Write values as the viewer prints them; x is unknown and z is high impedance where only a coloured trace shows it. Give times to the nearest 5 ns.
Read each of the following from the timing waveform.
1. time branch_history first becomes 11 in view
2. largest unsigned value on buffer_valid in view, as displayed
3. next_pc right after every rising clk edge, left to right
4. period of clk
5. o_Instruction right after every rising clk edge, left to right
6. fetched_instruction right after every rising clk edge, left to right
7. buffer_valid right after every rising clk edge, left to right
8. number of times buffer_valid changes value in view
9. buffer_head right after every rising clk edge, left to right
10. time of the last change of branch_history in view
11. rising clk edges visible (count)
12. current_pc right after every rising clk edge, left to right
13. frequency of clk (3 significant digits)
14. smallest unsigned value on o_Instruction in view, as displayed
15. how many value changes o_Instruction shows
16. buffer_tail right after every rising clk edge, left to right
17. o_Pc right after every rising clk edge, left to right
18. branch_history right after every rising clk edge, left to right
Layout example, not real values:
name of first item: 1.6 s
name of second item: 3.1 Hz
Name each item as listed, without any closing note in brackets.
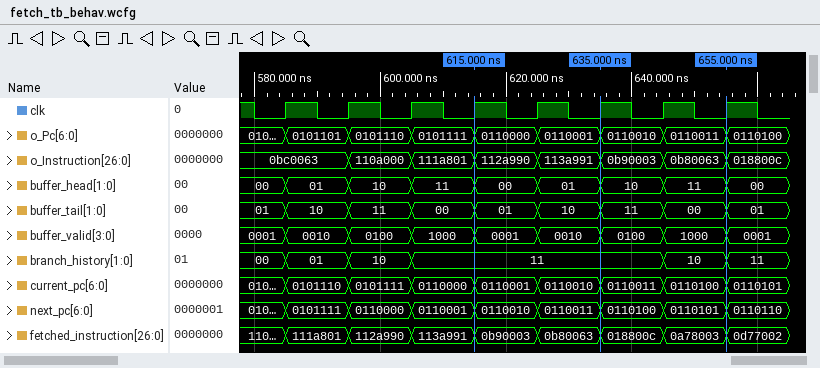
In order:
time branch_history first becomes 11 in view: 605 ns
largest unsigned value on buffer_valid in view, as displayed: 1000
next_pc right after every rising clk edge, left to right: 0101111, 0110000, 0110001, 0110010, 0110011, 0110100, 0110101, 0110110
period of clk: 10 ns
o_Instruction right after every rising clk edge, left to right: 0bc0063, 110a000, 111a801, 112a990, 113a991, 0b90003, 0b80063, 018800c
fetched_instruction right after every rising clk edge, left to right: 111a801, 112a990, 113a991, 0b90003, 0b80063, 018800c, 0a78003, 0d77002
buffer_valid right after every rising clk edge, left to right: 0010, 0100, 1000, 0001, 0010, 0100, 1000, 0001
number of times buffer_valid changes value in view: 8
buffer_head right after every rising clk edge, left to right: 01, 10, 11, 00, 01, 10, 11, 00
time of the last change of branch_history in view: 655 ns
rising clk edges visible: 8
current_pc right after every rising clk edge, left to right: 0101110, 0101111, 0110000, 0110001, 0110010, 0110011, 0110100, 0110101
frequency of clk: 100 MHz
smallest unsigned value on o_Instruction in view, as displayed: 018800c
how many value changes o_Instruction shows: 7
buffer_tail right after every rising clk edge, left to right: 10, 11, 00, 01, 10, 11, 00, 01
o_Pc right after every rising clk edge, left to right: 0101101, 0101110, 0101111, 0110000, 0110001, 0110010, 0110011, 0110100
branch_history right after every rising clk edge, left to right: 01, 10, 11, 11, 11, 11, 10, 11
